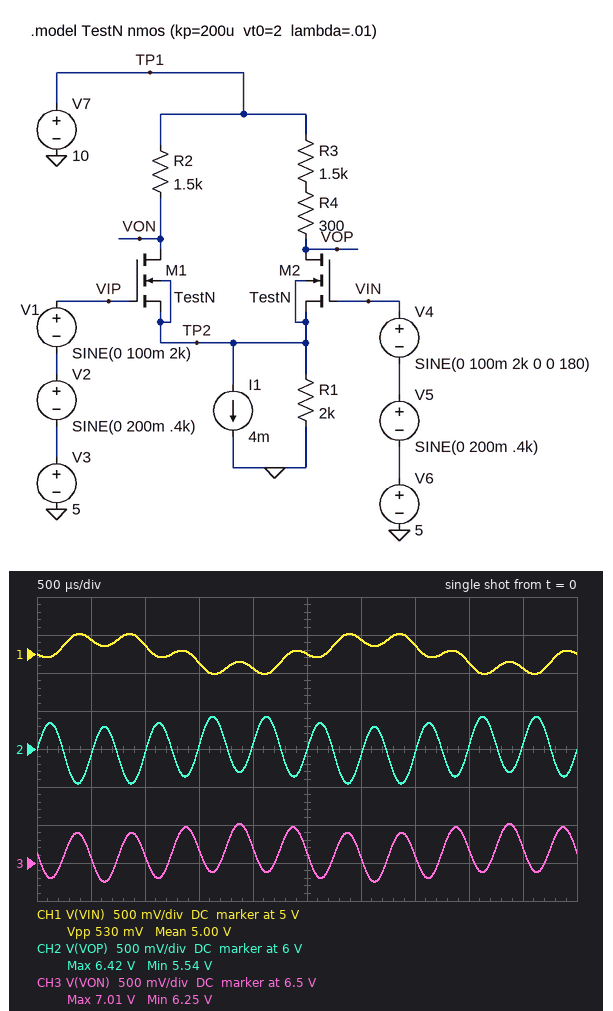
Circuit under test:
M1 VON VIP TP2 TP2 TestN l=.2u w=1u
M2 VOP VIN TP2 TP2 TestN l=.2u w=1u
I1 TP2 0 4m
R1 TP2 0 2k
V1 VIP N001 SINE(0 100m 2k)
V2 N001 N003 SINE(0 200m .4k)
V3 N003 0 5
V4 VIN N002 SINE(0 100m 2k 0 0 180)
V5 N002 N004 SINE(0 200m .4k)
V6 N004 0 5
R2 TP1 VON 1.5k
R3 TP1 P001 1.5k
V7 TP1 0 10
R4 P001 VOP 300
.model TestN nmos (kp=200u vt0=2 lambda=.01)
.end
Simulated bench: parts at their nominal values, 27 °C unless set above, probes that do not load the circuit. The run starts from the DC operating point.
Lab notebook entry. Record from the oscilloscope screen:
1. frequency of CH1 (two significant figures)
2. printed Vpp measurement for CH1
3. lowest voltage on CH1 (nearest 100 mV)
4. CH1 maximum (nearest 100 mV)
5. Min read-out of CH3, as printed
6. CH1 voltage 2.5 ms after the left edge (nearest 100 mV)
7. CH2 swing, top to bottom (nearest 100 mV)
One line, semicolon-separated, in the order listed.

400 Hz; 530 mV; 4.7 V; 5.3 V; 6.25 V; 5.0 V; 900 mV
